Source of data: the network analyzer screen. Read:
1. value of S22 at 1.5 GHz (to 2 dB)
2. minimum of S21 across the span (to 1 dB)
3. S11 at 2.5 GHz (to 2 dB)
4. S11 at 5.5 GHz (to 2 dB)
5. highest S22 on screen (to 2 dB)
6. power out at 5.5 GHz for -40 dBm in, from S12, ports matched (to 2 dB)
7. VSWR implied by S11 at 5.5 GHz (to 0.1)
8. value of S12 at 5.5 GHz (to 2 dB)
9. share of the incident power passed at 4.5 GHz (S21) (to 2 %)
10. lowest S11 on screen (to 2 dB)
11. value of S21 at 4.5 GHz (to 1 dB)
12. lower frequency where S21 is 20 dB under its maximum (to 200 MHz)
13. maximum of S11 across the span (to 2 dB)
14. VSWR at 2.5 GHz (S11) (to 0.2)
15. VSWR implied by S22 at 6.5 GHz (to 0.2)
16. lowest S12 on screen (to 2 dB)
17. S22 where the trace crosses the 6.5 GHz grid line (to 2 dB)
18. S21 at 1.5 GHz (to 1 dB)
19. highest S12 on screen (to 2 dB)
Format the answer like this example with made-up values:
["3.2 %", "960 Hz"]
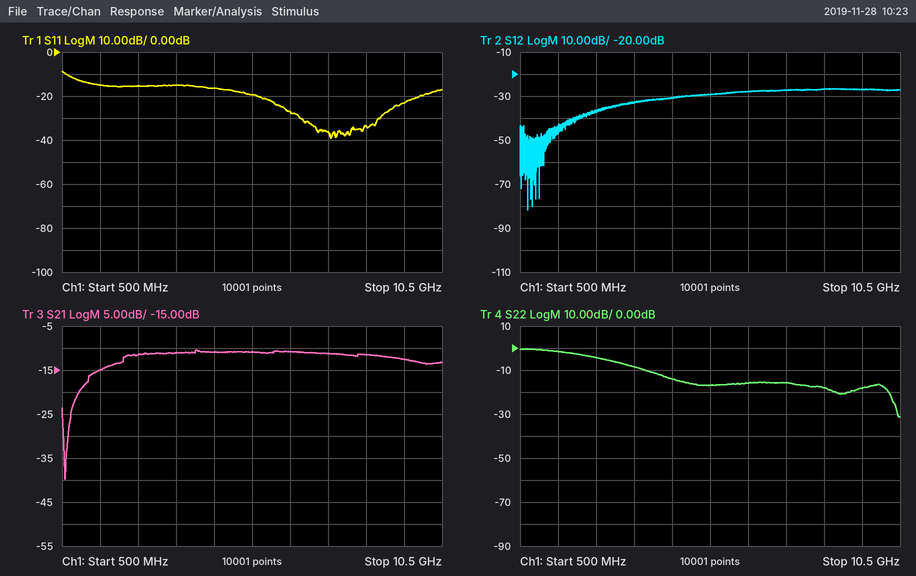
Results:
["-2 dB", "-40 dB", "-16 dB", "-20 dB", "0 dB", "-70 dBm", "1.2", "-30 dB", "8 %", "-40 dB", "-11 dB", "600 MHz", "-8 dB", "1.4", "1.4", "-82 dB", "-16 dB", "-15 dB", "-26 dB"]
